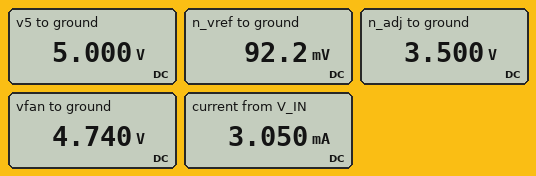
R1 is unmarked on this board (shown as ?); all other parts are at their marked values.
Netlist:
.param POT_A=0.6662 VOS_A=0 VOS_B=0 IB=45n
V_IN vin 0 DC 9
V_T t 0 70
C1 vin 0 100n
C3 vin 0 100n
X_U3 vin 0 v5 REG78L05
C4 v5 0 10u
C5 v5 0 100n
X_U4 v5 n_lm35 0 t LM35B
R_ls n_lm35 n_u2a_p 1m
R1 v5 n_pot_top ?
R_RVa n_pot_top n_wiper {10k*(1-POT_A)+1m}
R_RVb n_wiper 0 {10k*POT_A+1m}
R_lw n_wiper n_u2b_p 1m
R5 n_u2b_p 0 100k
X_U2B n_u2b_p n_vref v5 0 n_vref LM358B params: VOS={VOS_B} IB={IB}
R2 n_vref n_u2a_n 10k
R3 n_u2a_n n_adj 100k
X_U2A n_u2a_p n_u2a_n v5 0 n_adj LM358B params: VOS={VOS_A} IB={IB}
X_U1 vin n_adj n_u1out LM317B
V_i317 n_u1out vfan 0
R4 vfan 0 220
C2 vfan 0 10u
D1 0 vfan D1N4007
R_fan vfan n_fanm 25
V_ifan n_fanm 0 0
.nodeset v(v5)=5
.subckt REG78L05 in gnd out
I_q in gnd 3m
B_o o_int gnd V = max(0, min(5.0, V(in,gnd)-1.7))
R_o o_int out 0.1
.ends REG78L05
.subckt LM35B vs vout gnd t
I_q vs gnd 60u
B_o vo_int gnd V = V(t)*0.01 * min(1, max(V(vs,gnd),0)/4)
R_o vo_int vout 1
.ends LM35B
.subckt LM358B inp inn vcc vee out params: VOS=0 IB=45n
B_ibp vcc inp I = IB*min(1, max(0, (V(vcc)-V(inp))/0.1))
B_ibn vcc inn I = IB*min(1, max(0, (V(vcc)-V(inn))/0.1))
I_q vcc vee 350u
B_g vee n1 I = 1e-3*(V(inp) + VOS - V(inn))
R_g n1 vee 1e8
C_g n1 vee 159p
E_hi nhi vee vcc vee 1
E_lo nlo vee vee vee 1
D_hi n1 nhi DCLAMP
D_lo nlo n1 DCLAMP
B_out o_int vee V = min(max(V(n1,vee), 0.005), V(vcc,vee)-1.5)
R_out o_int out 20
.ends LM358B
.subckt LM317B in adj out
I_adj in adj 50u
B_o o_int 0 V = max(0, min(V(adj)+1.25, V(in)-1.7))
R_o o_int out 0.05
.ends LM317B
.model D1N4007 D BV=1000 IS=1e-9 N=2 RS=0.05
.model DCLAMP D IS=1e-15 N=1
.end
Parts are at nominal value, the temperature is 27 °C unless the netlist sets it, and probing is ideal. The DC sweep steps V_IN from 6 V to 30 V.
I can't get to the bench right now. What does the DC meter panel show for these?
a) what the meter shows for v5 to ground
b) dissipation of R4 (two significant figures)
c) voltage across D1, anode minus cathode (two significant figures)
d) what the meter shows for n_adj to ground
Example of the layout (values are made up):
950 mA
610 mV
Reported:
5.000 V
100 mW
-4.7 V
3.500 V
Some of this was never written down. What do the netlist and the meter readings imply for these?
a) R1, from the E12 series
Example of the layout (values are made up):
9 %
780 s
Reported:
330 kΩ
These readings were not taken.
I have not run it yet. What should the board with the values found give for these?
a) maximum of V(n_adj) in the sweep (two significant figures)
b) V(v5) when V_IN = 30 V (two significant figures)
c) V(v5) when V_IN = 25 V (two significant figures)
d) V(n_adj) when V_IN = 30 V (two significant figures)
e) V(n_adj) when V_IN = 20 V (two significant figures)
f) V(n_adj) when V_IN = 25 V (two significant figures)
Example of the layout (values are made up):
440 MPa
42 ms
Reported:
3.5 V
5.0 V
5.0 V
3.5 V
3.5 V
3.5 V
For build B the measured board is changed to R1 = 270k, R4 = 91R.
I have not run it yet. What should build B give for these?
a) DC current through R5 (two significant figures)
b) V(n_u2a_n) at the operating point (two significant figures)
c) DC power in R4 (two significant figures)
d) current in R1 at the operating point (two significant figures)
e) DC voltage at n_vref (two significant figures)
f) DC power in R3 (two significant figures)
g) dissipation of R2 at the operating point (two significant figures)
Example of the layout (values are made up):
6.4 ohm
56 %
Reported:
1.1 µA
420 mV
250 mW
18 µA
110 mV
95 µW
9.5 µW
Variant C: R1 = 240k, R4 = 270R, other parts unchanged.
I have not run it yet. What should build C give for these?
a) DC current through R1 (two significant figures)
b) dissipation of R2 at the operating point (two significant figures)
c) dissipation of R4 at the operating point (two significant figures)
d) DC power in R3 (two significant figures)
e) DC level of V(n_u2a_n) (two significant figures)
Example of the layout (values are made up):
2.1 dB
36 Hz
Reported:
20 µA
9.4 µW
83 mW
94 µW
430 mV
